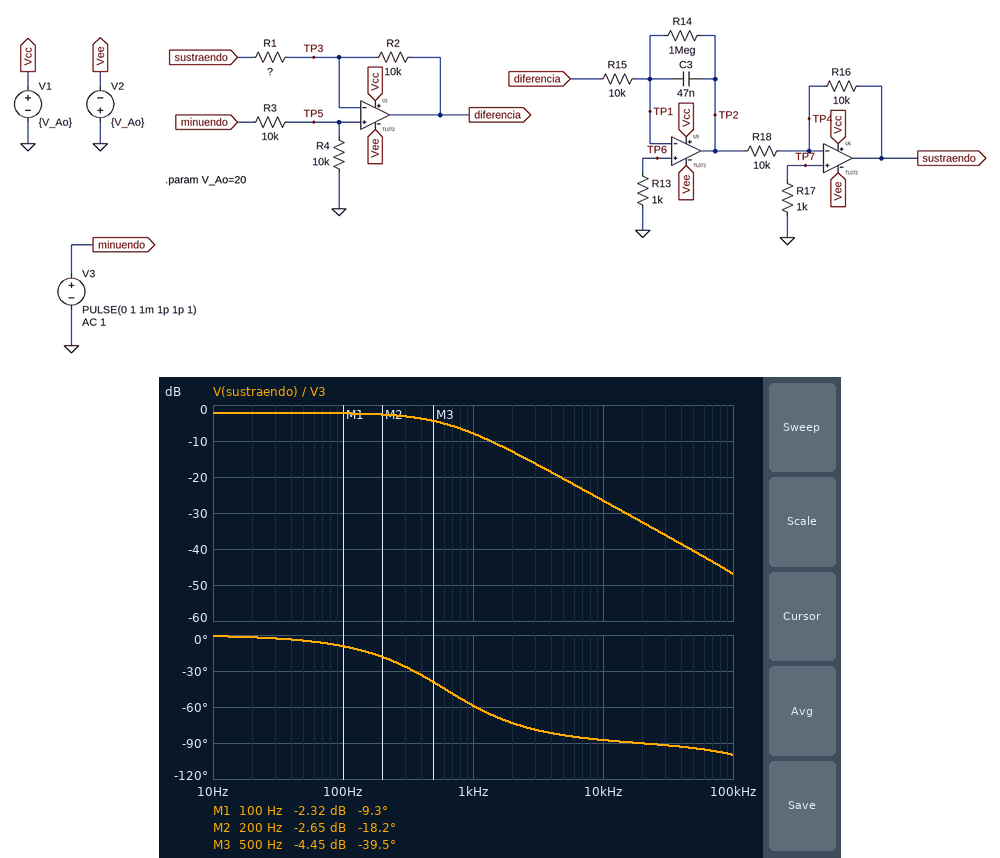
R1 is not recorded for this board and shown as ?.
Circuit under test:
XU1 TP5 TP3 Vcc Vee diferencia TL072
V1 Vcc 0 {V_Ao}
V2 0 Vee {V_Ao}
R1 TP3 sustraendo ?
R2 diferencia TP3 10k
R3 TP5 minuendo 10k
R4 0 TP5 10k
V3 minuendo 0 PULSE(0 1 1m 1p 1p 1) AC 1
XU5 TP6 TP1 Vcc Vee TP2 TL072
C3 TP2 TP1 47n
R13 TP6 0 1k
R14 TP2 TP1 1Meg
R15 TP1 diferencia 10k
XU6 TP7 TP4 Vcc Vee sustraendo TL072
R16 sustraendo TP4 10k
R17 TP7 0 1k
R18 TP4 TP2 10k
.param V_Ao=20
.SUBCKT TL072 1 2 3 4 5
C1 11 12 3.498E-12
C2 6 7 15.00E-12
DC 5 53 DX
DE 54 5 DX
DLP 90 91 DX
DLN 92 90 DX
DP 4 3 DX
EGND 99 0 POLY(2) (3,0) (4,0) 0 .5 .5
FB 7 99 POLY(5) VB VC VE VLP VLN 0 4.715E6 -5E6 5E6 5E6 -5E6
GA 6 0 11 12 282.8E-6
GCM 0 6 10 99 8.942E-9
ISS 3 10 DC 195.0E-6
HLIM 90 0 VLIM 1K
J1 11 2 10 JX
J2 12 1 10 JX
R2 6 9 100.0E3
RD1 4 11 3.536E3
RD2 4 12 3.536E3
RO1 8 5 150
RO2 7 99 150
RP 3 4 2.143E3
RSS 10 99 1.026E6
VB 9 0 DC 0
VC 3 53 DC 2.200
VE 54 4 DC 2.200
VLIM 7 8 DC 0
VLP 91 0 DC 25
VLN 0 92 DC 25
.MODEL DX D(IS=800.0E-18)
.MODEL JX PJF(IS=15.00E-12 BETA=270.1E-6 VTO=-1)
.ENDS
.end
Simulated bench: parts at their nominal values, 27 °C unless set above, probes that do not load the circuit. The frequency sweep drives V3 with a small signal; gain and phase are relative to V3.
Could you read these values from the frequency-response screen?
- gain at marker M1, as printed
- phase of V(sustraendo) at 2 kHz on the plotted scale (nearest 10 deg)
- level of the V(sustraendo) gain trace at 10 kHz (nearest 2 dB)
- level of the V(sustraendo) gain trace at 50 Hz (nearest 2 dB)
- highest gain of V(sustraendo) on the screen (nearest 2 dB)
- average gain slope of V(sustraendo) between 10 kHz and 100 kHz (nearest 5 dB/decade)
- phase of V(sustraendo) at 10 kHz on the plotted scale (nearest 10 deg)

-2.32 dB
-70 deg
-26 dB
-2 dB
-2 dB
-20 dB/decade
-90 deg
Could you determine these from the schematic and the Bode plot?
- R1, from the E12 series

5.6 kΩ
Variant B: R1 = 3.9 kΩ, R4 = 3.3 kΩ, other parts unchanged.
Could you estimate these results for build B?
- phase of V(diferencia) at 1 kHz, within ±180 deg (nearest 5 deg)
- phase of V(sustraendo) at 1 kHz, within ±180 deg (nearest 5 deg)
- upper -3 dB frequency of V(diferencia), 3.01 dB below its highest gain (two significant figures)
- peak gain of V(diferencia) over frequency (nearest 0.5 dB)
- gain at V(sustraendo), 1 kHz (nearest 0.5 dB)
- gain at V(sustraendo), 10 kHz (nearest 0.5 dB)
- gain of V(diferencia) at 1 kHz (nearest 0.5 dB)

40 deg
-50 deg
1.1 MHz
-1.0 dB
-13.0 dB
-30.5 dB
-3.5 dB
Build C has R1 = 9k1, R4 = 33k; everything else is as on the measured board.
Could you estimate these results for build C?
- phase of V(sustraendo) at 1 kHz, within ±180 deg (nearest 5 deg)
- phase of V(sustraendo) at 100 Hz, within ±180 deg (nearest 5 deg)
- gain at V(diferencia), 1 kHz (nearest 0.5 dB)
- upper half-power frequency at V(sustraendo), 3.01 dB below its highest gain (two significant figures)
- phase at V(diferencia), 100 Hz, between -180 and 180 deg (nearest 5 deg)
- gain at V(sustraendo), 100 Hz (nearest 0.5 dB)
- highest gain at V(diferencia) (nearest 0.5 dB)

-70 deg
-15 deg
3.5 dB
380 Hz
75 deg
3.0 dB
4.0 dB
